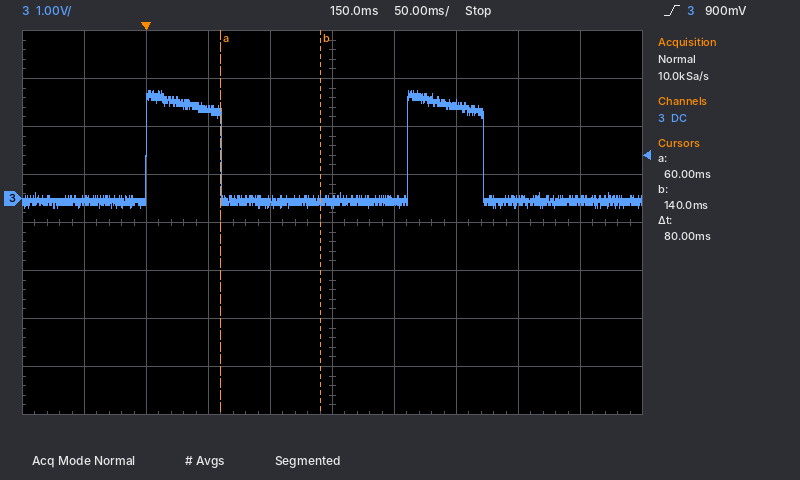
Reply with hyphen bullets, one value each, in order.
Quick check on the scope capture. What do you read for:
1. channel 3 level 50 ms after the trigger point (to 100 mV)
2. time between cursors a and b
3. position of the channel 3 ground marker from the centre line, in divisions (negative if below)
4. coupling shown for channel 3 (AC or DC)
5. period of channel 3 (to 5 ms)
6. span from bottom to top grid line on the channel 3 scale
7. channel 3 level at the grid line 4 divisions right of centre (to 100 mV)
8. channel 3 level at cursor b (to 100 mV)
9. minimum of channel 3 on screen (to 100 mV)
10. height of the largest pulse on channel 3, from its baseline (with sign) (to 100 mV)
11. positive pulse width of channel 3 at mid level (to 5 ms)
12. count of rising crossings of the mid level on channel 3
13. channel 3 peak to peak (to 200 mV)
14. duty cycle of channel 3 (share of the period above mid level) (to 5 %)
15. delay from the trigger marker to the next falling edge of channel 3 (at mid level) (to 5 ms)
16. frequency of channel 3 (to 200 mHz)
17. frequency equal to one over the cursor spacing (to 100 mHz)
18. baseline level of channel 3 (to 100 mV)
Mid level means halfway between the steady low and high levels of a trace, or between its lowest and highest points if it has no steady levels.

- 1.9 V
- 80 ms
- +0.5 div
- DC
- 210 ms
- 8 V
- 0.0 V
- 0.0 V
- -200 mV
- +2.3 V
- 60 ms
- 2
- 2.4 V
- 30 %
- 60 ms
- 4.8 Hz
- 12.5 Hz
- -100 mV
